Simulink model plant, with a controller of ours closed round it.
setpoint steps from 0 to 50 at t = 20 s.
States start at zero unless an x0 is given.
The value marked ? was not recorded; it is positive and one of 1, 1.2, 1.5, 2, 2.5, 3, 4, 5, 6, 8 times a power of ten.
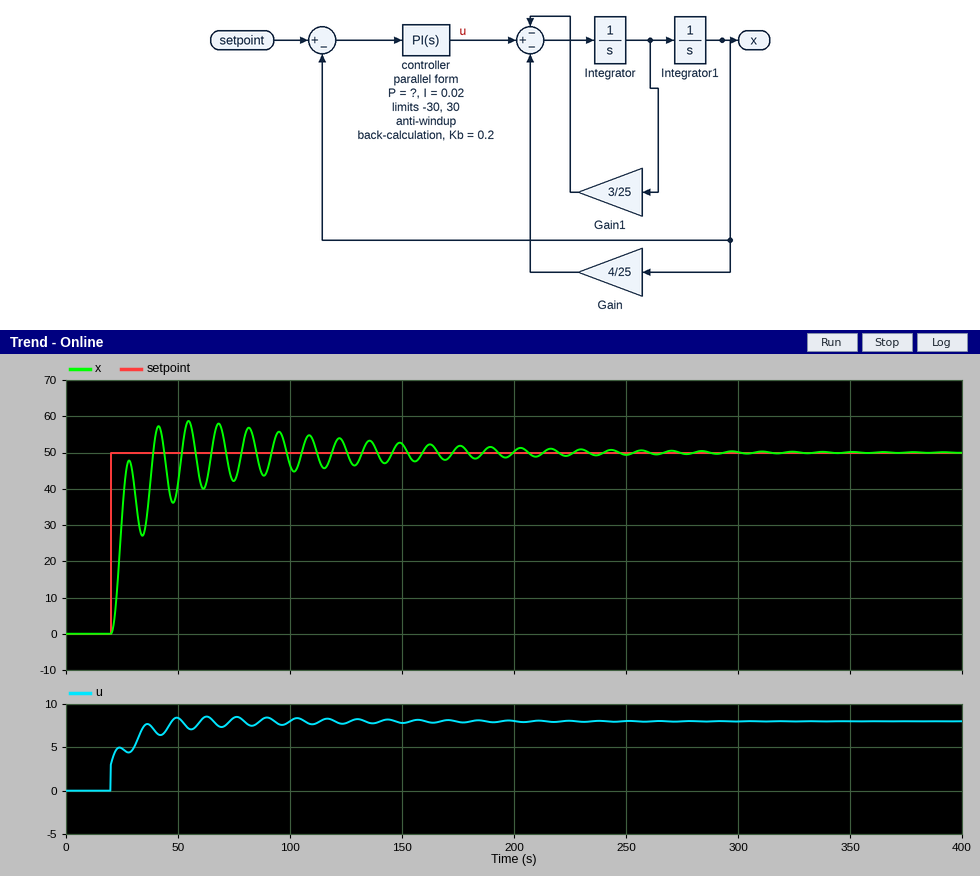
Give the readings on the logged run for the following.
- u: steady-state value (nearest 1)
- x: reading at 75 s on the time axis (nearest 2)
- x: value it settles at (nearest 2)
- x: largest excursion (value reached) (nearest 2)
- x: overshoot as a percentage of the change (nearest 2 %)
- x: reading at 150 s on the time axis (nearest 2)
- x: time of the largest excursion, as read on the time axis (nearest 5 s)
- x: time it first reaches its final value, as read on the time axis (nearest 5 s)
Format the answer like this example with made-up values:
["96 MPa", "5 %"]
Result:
["8", "42", "50", "58", "18 %", "52", "55 s", "40 s"]
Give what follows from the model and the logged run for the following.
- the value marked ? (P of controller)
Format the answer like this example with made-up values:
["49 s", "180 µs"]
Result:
["0.06"]
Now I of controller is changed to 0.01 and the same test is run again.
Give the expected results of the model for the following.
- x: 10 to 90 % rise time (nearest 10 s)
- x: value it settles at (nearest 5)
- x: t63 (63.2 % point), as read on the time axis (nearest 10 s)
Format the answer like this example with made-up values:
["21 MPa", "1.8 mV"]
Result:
["30 s", "50", "30 s"]
